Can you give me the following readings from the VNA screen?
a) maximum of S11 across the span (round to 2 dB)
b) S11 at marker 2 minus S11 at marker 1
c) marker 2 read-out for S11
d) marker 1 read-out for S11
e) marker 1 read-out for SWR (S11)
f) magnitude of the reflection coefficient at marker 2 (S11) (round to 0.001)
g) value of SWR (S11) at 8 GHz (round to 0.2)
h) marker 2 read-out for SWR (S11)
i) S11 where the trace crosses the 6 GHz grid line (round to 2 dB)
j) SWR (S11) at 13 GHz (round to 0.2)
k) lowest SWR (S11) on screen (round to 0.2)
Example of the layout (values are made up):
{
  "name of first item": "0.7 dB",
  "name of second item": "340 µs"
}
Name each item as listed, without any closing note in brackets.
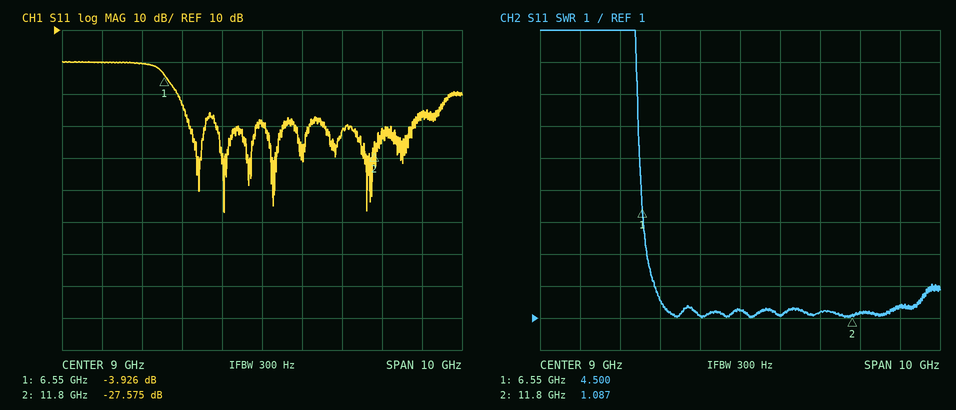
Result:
{
  "maximum of S11 across the span": "0 dB",
  "S11 at marker 2 minus S11 at marker 1": "-23.649 dB",
  "marker 2 read-out for S11": "-27.575 dB",
  "marker 1 read-out for S11": "-3.926 dB",
  "marker 1 read-out for SWR": "4.500",
  "magnitude of the reflection coefficient at marker 2 (S11)": "0.042",
  "value of SWR (S11) at 8 GHz": "1.0",
  "marker 2 read-out for SWR": "1.087",
  "S11 where the trace crosses the 6 GHz grid line": "0 dB",
  "SWR (S11) at 13 GHz": "1.4",
  "lowest SWR (S11) on screen": "1.0"
}
